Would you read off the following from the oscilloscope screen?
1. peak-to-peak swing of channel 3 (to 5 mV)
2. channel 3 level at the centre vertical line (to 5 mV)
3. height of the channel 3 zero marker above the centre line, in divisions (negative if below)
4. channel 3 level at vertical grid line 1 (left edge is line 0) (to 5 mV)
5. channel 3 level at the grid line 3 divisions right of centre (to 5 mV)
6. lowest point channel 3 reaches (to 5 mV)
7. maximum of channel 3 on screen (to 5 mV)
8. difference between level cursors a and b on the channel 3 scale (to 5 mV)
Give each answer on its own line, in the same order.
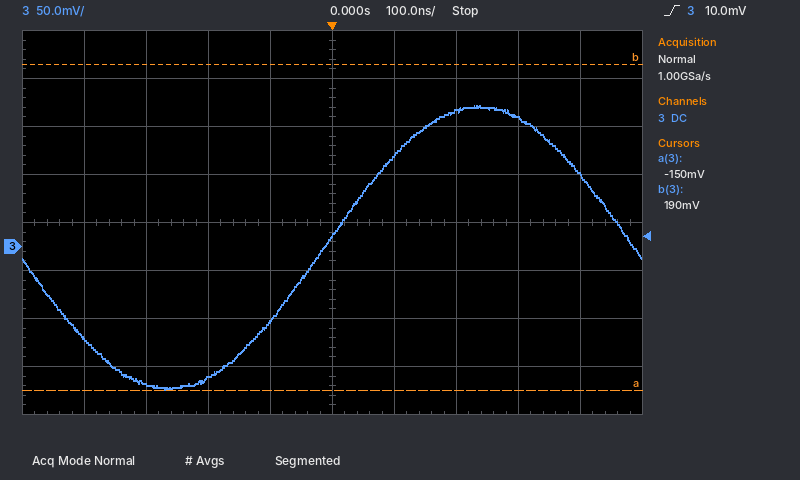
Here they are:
295 mV
10 mV
-0.5 div
-95 mV
135 mV
-150 mV
145 mV
340 mV
